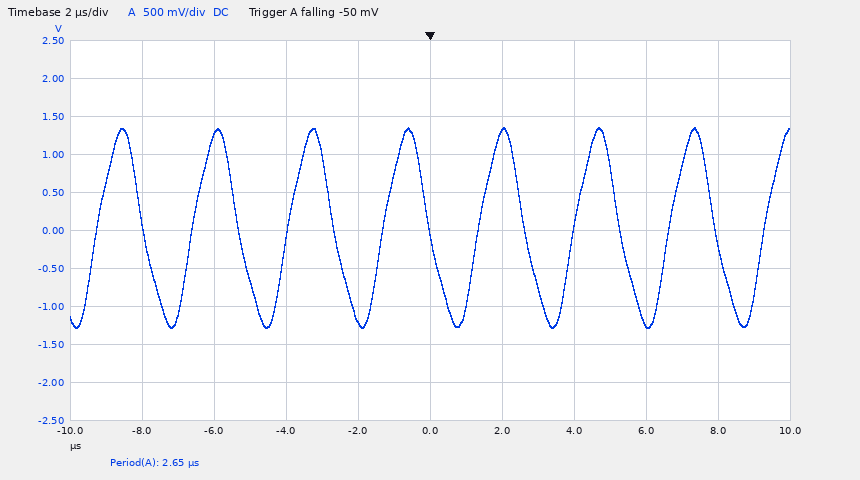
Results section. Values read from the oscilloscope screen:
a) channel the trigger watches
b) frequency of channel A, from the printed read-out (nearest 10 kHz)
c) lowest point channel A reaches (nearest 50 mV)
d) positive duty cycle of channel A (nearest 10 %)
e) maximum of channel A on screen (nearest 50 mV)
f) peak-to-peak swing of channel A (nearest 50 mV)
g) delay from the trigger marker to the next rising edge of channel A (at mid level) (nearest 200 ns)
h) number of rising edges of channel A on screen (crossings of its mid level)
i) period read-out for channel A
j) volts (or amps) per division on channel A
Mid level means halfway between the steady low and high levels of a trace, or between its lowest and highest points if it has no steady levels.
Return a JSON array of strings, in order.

["channel A", "380 kHz", "-1.30 V", "50 %", "1.35 V", "2.65 V", "1.4 µs", "8", "2.65 µs", "500 mV"]
